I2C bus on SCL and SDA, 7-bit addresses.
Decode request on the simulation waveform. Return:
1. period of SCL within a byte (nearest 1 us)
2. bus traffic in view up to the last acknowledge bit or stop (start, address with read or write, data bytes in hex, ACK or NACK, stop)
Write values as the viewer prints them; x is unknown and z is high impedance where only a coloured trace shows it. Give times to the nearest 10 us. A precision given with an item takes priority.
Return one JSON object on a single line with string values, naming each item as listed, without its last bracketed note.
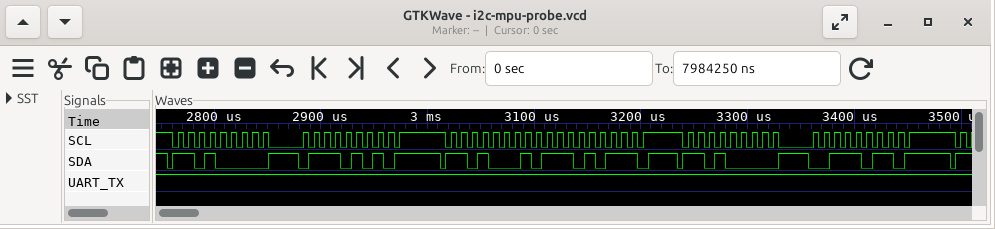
{"period of SCL within a byte": "10 us", "bus traffic in view up to the last acknowledge bit or stop": "start, address 68 write ACK, 75 ACK, repeated start, address 68 read ACK, EB NACK, stop, start, address 68 write ACK, 3B ACK"}
